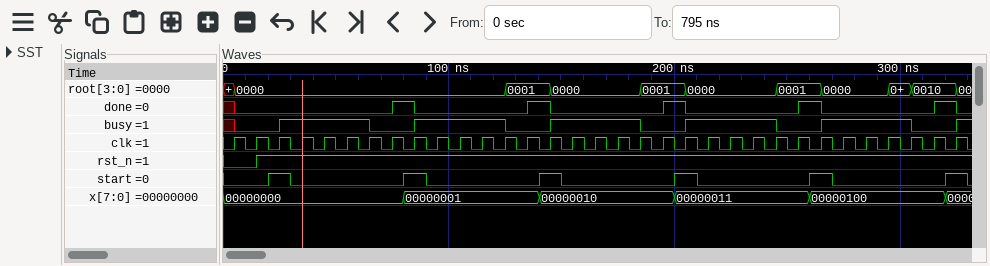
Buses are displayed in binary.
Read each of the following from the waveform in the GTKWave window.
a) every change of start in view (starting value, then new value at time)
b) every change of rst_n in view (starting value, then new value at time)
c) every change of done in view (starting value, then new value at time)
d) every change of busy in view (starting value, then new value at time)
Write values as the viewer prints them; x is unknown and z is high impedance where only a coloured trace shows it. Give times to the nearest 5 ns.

0, 1 at 20 ns, 0 at 30 ns, 1 at 80 ns, 0 at 90 ns, 1 at 140 ns, 0 at 150 ns, 1 at 200 ns, 0 at 210 ns, 1 at 260 ns, 0 at 270 ns, 1 at 320 ns, 0 at 330 ns
0, 1 at 15 ns
x, 0 at 5 ns, 1 at 75 ns, 0 at 85 ns, 1 at 135 ns, 0 at 145 ns, 1 at 195 ns, 0 at 205 ns, 1 at 255 ns, 0 at 265 ns, 1 at 315 ns, 0 at 325 ns
x, 0 at 5 ns, 1 at 25 ns, 0 at 65 ns, 1 at 85 ns, 0 at 125 ns, 1 at 145 ns, 0 at 185 ns, 1 at 205 ns, 0 at 245 ns, 1 at 265 ns, 0 at 305 ns, 1 at 325 ns
